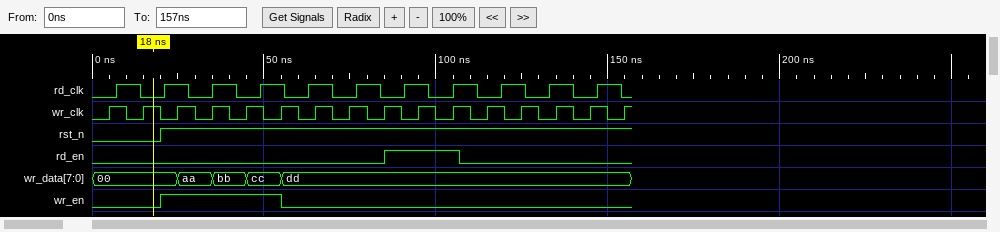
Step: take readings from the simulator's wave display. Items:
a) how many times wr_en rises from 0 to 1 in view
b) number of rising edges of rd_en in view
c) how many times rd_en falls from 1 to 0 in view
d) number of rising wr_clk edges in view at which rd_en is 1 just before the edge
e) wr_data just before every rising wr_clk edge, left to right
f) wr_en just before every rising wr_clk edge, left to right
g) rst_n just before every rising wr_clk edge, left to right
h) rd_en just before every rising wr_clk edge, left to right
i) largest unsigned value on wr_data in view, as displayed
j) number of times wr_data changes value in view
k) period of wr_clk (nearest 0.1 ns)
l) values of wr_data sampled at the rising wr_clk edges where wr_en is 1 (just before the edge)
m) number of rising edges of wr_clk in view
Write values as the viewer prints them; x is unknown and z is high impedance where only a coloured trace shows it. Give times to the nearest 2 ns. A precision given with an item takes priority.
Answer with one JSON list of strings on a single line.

["1", "1", "1", "2", "00, 00, 00, aa, bb, cc, dd, dd, dd, dd, dd, dd, dd, dd, dd, dd", "0 0 1 1 1 1 0 0 0 0 0 0 0 0 0 0", "0 0 1 1 1 1 1 1 1 1 1 1 1 1 1 1", "0 0 0 0 0 0 0 0 0 1 1 0 0 0 0 0", "dd", "4", "10 ns", "00, aa, bb, cc", "16"]
